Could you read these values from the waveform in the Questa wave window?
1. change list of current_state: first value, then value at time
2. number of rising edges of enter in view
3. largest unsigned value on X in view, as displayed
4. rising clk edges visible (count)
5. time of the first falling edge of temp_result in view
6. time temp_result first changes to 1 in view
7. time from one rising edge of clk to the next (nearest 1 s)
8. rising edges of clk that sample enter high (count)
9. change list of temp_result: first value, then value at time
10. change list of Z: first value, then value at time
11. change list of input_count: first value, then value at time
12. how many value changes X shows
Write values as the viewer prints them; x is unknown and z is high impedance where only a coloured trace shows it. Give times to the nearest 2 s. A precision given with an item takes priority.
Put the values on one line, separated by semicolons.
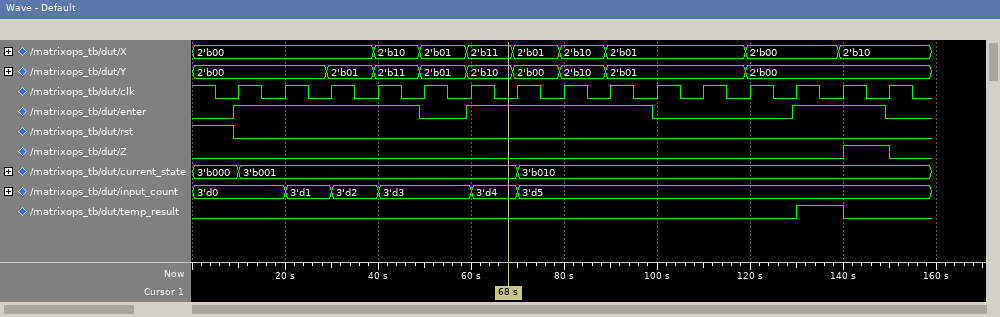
3'b000, 3'b001 at 10 s, 3'b010 at 70 s; 3; 2'b11; 15; 140 s; 130 s; 10 s; 10; 0, 1 at 130 s, 0 at 140 s; 0, 1 at 140 s, 0 at 150 s; 3'd0, 3'd1 at 20 s, 3'd2 at 30 s, 3'd3 at 40 s, 3'd4 at 60 s, 3'd5 at 70 s; 8
